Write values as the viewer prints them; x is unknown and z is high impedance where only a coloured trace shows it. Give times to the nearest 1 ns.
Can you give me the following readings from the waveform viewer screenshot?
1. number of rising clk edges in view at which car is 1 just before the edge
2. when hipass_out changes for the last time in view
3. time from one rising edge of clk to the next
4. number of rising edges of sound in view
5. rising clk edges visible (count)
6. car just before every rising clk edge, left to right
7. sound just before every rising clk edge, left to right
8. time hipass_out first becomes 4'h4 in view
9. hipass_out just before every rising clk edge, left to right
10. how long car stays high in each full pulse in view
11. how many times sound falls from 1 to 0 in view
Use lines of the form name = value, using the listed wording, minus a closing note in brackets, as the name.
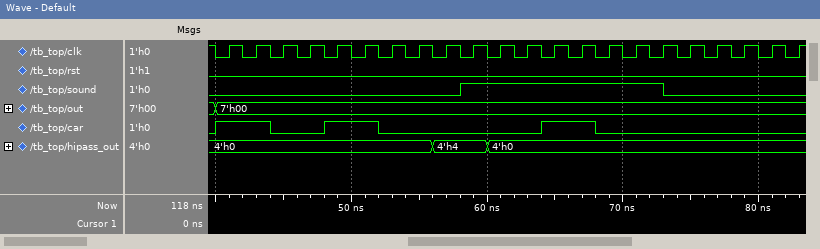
number of rising clk edges in view at which car is 1 just before the edge = 6
when hipass_out changes for the last time in view = 60 ns
time from one rising edge of clk to the next = 2 ns
number of rising edges of sound in view = 1
rising clk edges visible = 22
car just before every rising clk edge, left to right = 1 1 0 0 1 1 0 0 0 0 0 0 1 1 0 0 0 0 0 0 0 0
sound just before every rising clk edge, left to right = 0 0 0 0 0 0 0 0 0 1 1 1 1 1 1 1 1 0 0 0 0 0
time hipass_out first becomes 4'h4 in view = 56 ns
hipass_out just before every rising clk edge, left to right = 4'h0, 4'h0, 4'h0, 4'h0, 4'h0, 4'h0, 4'h0, 4'h0, 4'h4, 4'h4, 4'h0, 4'h0, 4'h0, 4'h0, 4'h0, 4'h0, 4'h0, 4'h0, 4'h0, 4'h0, 4'h0, 4'h0
how long car stays high in each full pulse in view = 4 ns, 4 ns, 4 ns
how many times sound falls from 1 to 0 in view = 1
